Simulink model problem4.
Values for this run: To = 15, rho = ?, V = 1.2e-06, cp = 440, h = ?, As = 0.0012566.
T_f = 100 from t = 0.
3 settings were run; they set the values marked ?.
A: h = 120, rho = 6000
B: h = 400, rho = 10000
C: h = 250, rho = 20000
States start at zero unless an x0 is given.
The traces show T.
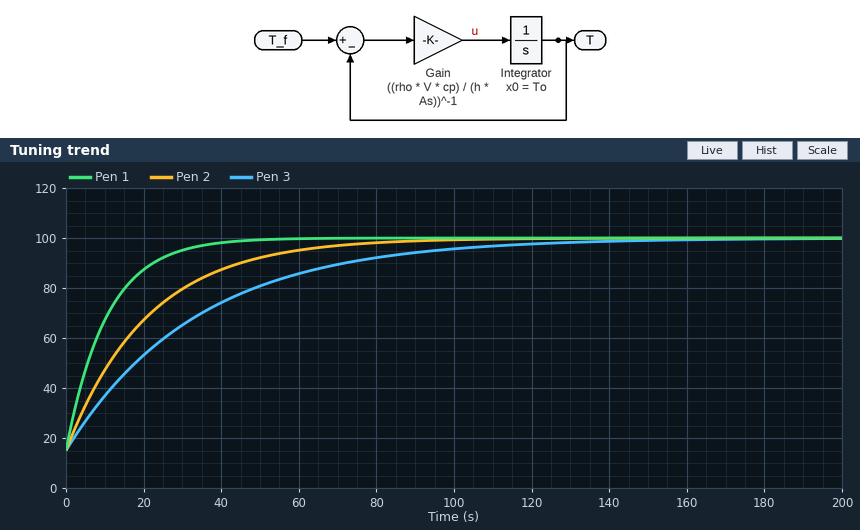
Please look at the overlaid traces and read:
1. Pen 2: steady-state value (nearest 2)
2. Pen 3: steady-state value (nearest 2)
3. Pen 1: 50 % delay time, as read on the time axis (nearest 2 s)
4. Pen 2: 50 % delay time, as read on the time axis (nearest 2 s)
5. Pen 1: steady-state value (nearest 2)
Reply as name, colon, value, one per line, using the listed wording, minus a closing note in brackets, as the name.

Pen 2: steady-state value: 100
Pen 3: steady-state value: 100
Pen 1: 50 % delay time, as read on the time axis: 8 s
Pen 2: 50 % delay time, as read on the time axis: 14 s
Pen 1: steady-state value: 100
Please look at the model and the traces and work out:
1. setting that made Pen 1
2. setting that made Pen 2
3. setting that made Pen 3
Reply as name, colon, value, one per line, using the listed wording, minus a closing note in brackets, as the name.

setting that made Pen 1: B
setting that made Pen 2: A
setting that made Pen 3: C
